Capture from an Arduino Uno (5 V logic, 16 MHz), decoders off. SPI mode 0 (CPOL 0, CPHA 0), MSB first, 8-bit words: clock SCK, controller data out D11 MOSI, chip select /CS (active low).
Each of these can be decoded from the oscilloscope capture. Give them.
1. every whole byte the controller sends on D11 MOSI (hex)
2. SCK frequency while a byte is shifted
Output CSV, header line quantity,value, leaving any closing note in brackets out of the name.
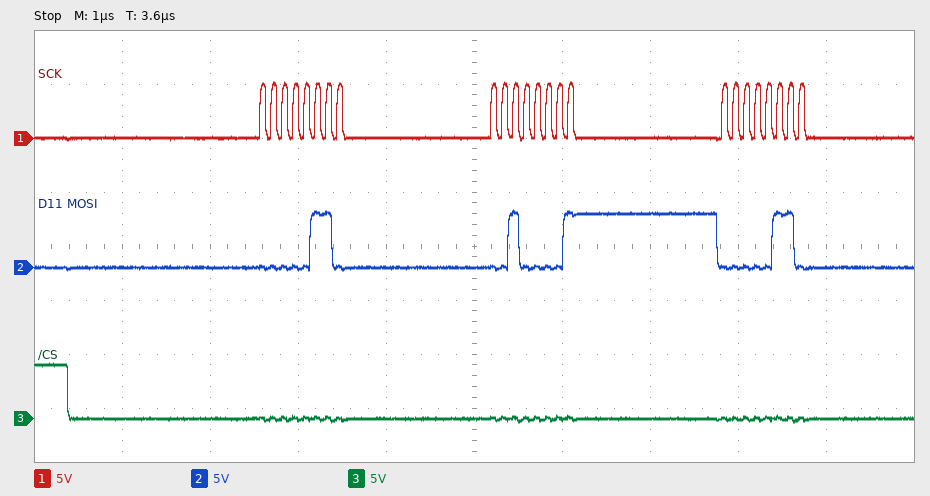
quantity,value
every whole byte the controller sends on D11 MOSI,06 21 06
SCK frequency while a byte is shifted,8 MHz
